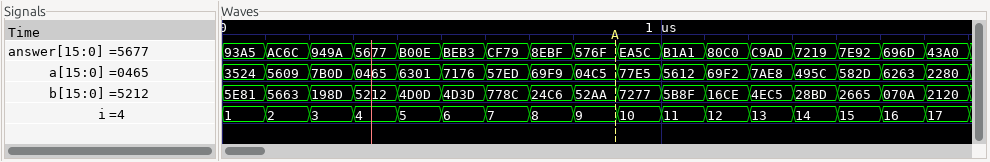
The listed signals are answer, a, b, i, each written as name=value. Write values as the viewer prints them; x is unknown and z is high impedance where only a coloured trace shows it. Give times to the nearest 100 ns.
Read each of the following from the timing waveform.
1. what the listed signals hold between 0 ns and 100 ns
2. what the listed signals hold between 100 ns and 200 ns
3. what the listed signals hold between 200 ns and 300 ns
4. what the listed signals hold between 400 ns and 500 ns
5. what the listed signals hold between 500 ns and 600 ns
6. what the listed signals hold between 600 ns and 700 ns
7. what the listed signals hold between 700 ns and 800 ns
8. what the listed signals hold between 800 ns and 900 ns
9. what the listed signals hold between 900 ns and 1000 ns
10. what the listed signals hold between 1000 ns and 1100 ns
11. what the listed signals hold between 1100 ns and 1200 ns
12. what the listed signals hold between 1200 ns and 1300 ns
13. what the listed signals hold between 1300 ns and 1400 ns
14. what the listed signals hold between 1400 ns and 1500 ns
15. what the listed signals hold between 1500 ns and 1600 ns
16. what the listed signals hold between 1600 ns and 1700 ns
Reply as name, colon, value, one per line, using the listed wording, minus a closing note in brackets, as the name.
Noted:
what the listed signals hold between 0 ns and 100 ns: answer=93A5, a=3524, b=5E81, i=1
what the listed signals hold between 100 ns and 200 ns: answer=AC6C, a=5609, b=5663, i=2
what the listed signals hold between 200 ns and 300 ns: answer=949A, a=7B0D, b=198D, i=3
what the listed signals hold between 400 ns and 500 ns: answer=B00E, a=6301, b=4D0D, i=5
what the listed signals hold between 500 ns and 600 ns: answer=BEB3, a=7176, b=4D3D, i=6
what the listed signals hold between 600 ns and 700 ns: answer=CF79, a=57ED, b=778C, i=7
what the listed signals hold between 700 ns and 800 ns: answer=8EBF, a=69F9, b=24C6, i=8
what the listed signals hold between 800 ns and 900 ns: answer=576F, a=04C5, b=52AA, i=9
what the listed signals hold between 900 ns and 1000 ns: answer=EA5C, a=77E5, b=7277, i=10
what the listed signals hold between 1000 ns and 1100 ns: answer=B1A1, a=5612, b=5B8F, i=11
what the listed signals hold between 1100 ns and 1200 ns: answer=80C0, a=69F2, b=16CE, i=12
what the listed signals hold between 1200 ns and 1300 ns: answer=C9AD, a=7AE8, b=4EC5, i=13
what the listed signals hold between 1300 ns and 1400 ns: answer=7219, a=495C, b=28BD, i=14
what the listed signals hold between 1400 ns and 1500 ns: answer=7E92, a=582D, b=2665, i=15
what the listed signals hold between 1500 ns and 1600 ns: answer=696D, a=6263, b=070A, i=16
what the listed signals hold between 1600 ns and 1700 ns: answer=43A0, a=2280, b=2120, i=17
